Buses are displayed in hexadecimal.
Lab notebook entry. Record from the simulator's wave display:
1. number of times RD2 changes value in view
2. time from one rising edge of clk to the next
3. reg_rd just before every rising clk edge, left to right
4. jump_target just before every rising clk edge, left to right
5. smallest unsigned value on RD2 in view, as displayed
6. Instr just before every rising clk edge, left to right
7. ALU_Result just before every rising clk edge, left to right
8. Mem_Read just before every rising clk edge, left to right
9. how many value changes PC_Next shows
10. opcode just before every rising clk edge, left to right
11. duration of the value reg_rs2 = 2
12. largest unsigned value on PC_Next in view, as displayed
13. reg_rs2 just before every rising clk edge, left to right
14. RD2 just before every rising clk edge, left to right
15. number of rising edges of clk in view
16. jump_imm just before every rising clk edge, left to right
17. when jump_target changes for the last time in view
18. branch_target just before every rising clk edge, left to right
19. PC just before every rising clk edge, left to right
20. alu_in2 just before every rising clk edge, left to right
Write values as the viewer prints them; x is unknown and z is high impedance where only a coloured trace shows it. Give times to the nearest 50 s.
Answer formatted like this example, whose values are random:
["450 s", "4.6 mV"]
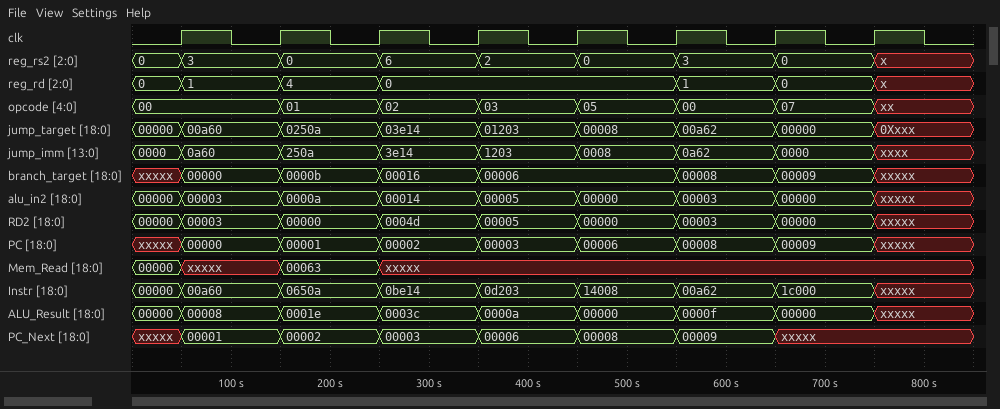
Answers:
["8", "100 s", "0, 1, 4, 0, 0, 0, 1, 0", "00000, 00a60, 0250a, 03e14, 01203, 00008, 00a62, 00000", "00000", "00000, 00a60, 0650a, 0be14, 0d203, 14008, 00a62, 1c000", "00000, 00008, 0001e, 0003c, 0000a, 00000, 0000f, 00000", "00000, xxxxx, 00063, xxxxx, xxxxx, xxxxx, xxxxx, xxxxx", "7", "00, 00, 01, 02, 03, 05, 00, 07", "100 s", "00009", "0, 3, 0, 6, 2, 0, 3, 0", "00000, 00003, 00000, 0004d, 00005, 00000, 00003, 00000", "8", "0000, 0a60, 250a, 3e14, 1203, 0008, 0a62, 0000", "750 s", "xxxxx, 00000, 0000b, 00016, 00006, 00006, 00008, 00009", "xxxxx, 00000, 00001, 00002, 00003, 00006, 00008, 00009", "00000, 00003, 0000a, 00014, 00005, 00000, 00003, 00000"]
